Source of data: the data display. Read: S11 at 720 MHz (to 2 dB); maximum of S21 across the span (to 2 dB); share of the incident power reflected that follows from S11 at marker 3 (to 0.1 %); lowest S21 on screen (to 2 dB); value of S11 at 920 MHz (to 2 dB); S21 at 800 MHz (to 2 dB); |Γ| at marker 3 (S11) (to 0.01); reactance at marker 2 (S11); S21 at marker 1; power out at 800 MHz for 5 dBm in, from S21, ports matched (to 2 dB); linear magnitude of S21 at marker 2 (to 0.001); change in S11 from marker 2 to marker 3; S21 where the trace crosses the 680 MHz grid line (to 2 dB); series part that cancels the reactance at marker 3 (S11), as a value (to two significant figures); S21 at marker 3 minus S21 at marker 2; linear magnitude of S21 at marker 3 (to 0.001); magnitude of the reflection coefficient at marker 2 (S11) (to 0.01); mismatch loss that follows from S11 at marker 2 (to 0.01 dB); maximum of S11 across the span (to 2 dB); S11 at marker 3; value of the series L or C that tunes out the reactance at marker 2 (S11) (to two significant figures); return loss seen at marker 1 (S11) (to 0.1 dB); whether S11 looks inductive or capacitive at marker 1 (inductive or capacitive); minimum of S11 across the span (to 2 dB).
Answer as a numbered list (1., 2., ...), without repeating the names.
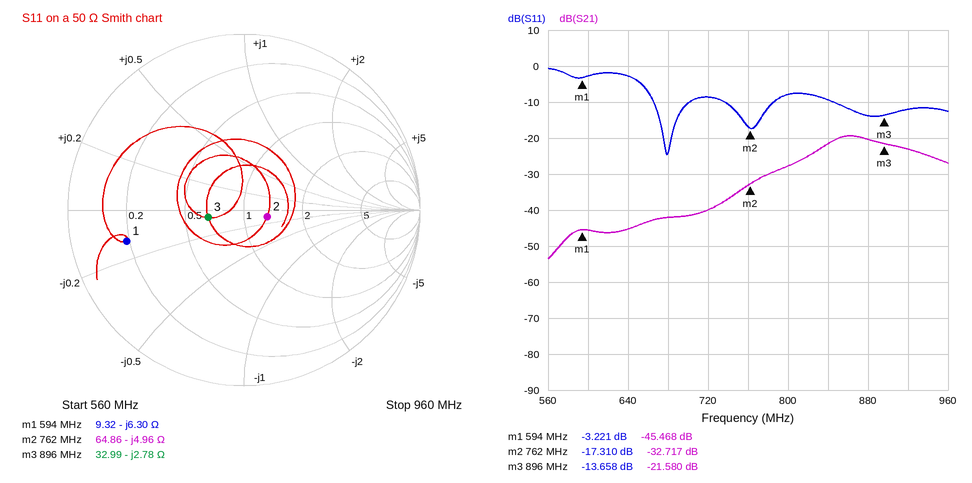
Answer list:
1. -8 dB
2. -20 dB
3. 4.3 %
4. -54 dB
5. -12 dB
6. -28 dB
7. 0.21
8. -4.96 Ω
9. -45.468 dB
10. -22 dBm
11. 0.023
12. 3.652 dB
13. -42 dB
14. 490 pH
15. 11.137 dB
16. 0.083
17. 0.14
18. 0.08 dB
19. 0 dB
20. -13.658 dB
21. 1.0 nH
22. 3.2 dB
23. capacitive
24. -24 dB
